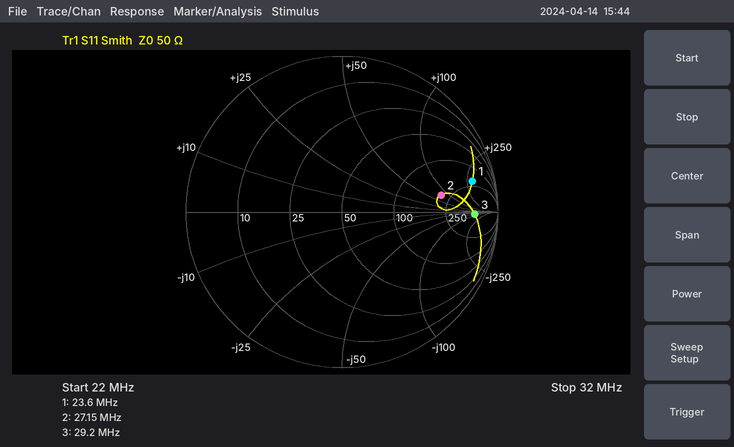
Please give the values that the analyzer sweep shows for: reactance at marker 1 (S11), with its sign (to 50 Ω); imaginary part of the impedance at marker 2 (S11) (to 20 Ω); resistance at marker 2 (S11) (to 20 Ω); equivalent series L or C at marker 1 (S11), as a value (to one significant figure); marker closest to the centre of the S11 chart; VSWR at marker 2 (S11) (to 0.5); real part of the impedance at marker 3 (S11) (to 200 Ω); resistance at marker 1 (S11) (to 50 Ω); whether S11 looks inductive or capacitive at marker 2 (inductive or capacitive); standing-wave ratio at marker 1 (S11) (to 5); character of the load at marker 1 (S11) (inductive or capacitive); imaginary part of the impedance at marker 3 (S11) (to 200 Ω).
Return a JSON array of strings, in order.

["+300 Ω", "+80 Ω", "200 Ω", "2 µH", "marker 2", "4.5", "600 Ω", "200 Ω", "inductive", "15", "inductive", "0 Ω"]
